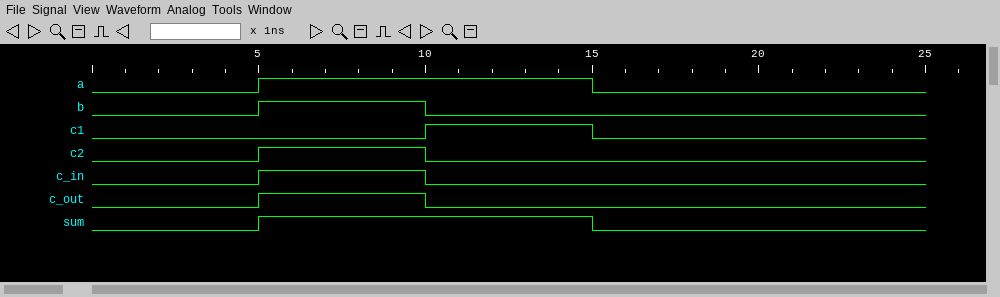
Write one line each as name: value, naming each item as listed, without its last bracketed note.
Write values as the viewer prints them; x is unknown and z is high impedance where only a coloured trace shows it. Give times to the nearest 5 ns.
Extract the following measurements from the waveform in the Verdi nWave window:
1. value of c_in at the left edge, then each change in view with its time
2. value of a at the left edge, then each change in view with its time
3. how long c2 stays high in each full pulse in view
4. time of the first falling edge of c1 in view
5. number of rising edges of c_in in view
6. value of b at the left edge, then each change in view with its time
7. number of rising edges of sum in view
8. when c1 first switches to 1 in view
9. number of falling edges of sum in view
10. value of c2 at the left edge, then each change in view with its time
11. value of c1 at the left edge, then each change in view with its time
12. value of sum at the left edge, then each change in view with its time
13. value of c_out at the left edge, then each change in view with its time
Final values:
value of c_in at the left edge, then each change in view with its time: 0, 1 at 5 ns, 0 at 10 ns
value of a at the left edge, then each change in view with its time: 0, 1 at 5 ns, 0 at 15 ns
how long c2 stays high in each full pulse in view: 5 ns
time of the first falling edge of c1 in view: 15 ns
number of rising edges of c_in in view: 1
value of b at the left edge, then each change in view with its time: 0, 1 at 5 ns, 0 at 10 ns
number of rising edges of sum in view: 1
when c1 first switches to 1 in view: 10 ns
number of falling edges of sum in view: 1
value of c2 at the left edge, then each change in view with its time: 0, 1 at 5 ns, 0 at 10 ns
value of c1 at the left edge, then each change in view with its time: 0, 1 at 10 ns, 0 at 15 ns
value of sum at the left edge, then each change in view with its time: 0, 1 at 5 ns, 0 at 15 ns
value of c_out at the left edge, then each change in view with its time: 0, 1 at 5 ns, 0 at 10 ns
